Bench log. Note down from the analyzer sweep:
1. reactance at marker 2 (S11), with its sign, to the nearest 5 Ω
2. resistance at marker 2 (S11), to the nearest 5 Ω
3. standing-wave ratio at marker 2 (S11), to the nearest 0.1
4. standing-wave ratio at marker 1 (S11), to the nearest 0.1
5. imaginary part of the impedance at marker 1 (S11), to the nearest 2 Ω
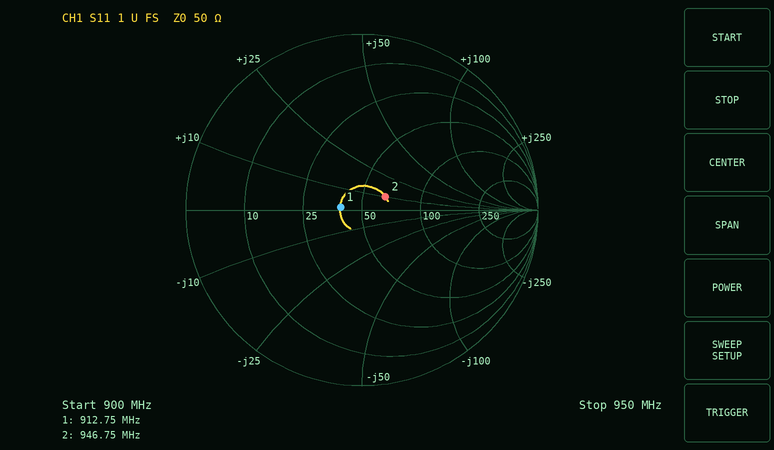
+10 Ω
65 Ω
1.4
1.3
+2 Ω
